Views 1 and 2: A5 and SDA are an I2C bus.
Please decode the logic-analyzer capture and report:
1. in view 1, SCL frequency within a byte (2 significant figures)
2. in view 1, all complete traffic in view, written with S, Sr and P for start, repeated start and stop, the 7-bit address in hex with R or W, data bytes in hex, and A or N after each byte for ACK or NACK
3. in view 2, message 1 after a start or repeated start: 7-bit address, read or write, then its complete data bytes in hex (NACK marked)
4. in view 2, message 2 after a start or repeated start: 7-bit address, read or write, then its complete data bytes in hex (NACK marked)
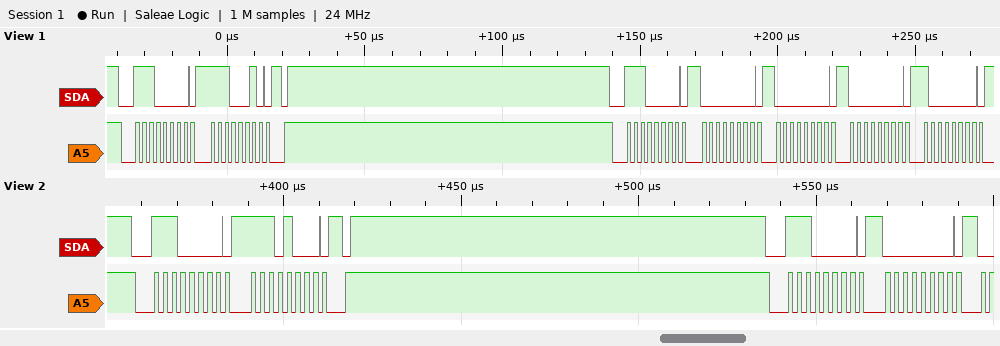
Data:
400 kHz
S 70W A E2 A P S 70W A 00 A 00 A 00 A 80 A
0x70 write: E8
0x70 write: 00
